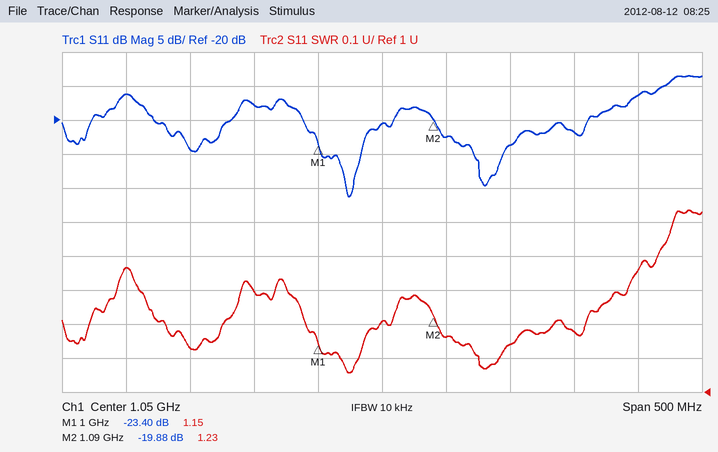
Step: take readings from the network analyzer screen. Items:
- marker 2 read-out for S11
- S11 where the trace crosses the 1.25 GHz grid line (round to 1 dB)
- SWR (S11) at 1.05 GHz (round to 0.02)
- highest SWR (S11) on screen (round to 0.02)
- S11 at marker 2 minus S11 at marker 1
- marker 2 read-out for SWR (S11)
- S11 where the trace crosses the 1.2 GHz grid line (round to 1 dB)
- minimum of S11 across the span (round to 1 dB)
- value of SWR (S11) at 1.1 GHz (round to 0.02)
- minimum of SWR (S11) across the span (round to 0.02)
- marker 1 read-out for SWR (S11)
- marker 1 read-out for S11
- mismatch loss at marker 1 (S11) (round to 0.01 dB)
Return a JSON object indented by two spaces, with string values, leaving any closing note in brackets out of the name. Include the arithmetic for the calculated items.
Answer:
{
  "marker 2 read-out for S11": "-19.88 dB",
  "S11 where the trace crosses the 1.25 GHz grid line": "-16 dB",
  "SWR (S11) at 1.05 GHz": "1.20",
  "highest SWR (S11) on screen": "1.54",
  "S11 at marker 2 minus S11 at marker 1": "-19.88 − (-23.4) = 3.52 dB",
  "marker 2 read-out for SWR": "1.23",
  "S11 where the trace crosses the 1.2 GHz grid line": "-22 dB",
  "minimum of S11 across the span": "-31 dB",
  "value of SWR (S11) at 1.1 GHz": "1.16",
  "minimum of SWR (S11) across the span": "1.06",
  "marker 1 read-out for SWR": "1.15",
  "marker 1 read-out for S11": "-23.40 dB",
  "mismatch loss at marker 1 (S11)": "−10 log10(1 − 10^(-23.4/10)) ≈ 0.02 dB"
}
